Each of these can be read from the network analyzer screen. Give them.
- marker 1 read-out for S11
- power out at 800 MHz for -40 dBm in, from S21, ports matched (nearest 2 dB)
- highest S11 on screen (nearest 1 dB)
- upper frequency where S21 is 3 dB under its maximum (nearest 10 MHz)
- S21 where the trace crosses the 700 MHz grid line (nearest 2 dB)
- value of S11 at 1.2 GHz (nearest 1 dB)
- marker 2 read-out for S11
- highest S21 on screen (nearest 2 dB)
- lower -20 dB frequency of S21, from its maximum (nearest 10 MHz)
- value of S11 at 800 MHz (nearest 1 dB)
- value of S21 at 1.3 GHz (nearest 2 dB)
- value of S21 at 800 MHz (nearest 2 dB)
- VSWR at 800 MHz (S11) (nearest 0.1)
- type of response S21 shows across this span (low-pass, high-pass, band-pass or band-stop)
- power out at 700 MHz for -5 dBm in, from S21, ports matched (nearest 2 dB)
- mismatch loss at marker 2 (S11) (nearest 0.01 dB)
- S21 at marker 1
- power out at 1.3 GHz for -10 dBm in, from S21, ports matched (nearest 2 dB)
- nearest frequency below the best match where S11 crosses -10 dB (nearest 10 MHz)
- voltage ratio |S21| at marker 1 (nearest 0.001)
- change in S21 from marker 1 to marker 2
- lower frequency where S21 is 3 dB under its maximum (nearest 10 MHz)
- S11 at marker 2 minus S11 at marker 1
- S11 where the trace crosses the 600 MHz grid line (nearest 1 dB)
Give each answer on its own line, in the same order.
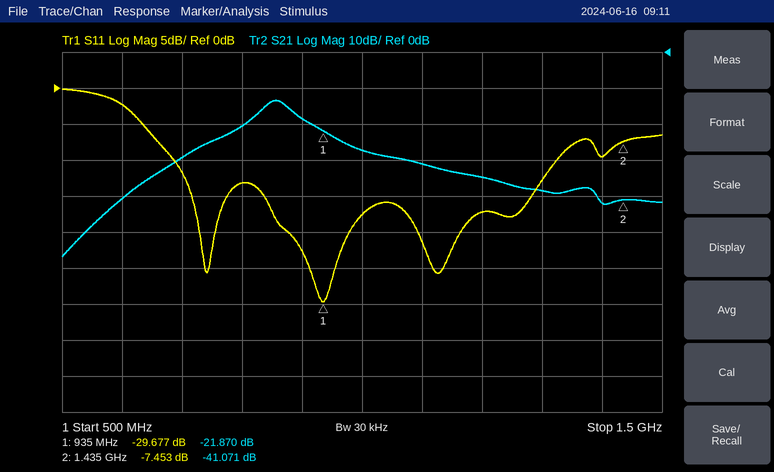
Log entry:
-29.677 dB
-60 dBm
0 dB
880 MHz
-30 dB
-17 dB
-7.453 dB
-14 dB
660 MHz
-13 dB
-38 dB
-20 dB
1.6
band-pass
-34 dBm
0.86 dB
-21.870 dB
-48 dBm
690 MHz
0.081
-19.201 dB
830 MHz
22.224 dB
-2 dB
